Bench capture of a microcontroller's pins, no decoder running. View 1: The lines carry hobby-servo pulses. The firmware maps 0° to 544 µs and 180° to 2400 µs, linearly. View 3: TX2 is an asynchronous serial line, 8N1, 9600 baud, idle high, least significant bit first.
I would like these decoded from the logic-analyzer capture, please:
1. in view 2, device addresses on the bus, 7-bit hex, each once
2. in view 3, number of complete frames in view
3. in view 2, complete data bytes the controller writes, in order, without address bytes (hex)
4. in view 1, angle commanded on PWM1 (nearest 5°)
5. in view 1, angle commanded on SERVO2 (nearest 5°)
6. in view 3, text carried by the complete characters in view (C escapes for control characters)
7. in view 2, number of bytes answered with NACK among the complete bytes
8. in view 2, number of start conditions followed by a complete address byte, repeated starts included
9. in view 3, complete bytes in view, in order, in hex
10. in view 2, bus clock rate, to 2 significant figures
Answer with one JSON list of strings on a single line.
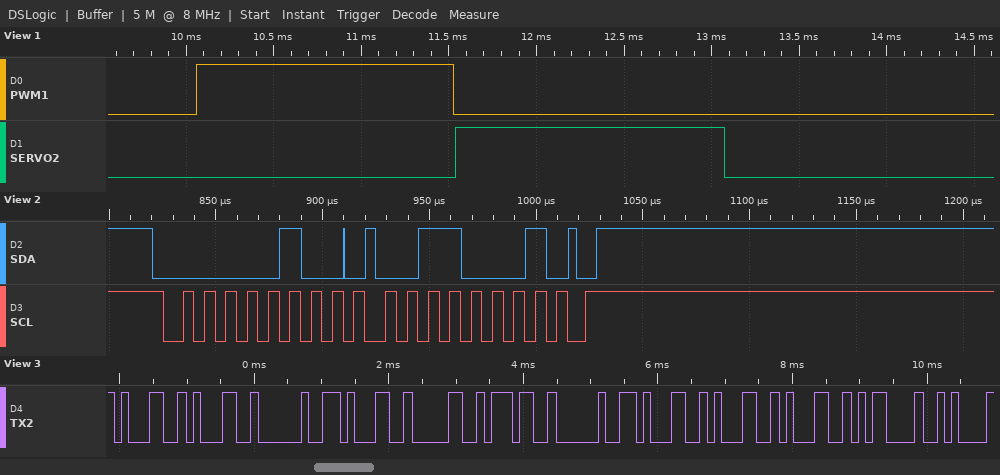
["0x02", "12", "31", "90°", "95°", "\"11 107 111\\r\\n\"", "0", "1", "31 31 20 31 30 37 20 31 31 31 0D 0A", "100 kHz"]
